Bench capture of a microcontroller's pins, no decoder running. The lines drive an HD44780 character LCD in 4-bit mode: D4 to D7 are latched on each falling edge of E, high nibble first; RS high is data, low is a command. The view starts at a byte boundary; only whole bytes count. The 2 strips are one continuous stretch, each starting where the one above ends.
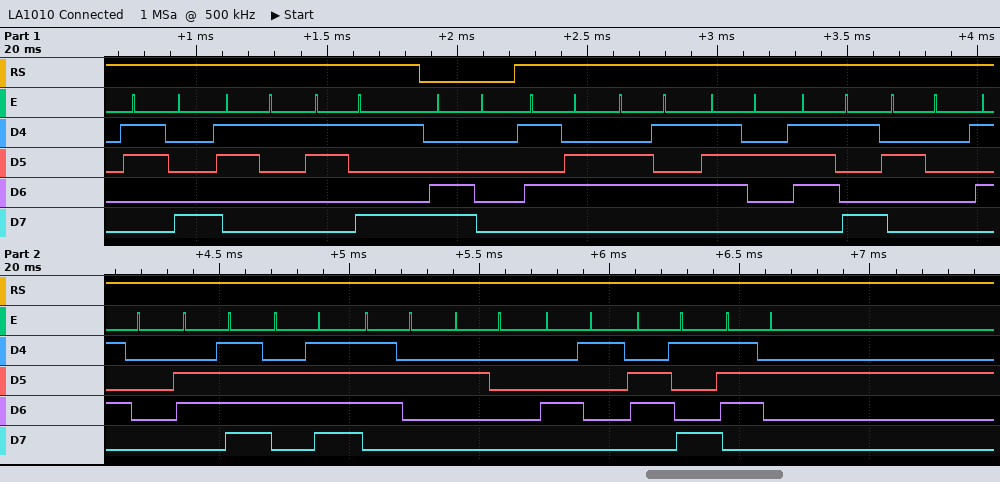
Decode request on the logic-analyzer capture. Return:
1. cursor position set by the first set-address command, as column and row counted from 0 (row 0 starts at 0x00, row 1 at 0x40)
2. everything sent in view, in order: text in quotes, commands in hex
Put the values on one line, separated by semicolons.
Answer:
column 0, row 1; "819" 0xC0 "Very Poor Air"
